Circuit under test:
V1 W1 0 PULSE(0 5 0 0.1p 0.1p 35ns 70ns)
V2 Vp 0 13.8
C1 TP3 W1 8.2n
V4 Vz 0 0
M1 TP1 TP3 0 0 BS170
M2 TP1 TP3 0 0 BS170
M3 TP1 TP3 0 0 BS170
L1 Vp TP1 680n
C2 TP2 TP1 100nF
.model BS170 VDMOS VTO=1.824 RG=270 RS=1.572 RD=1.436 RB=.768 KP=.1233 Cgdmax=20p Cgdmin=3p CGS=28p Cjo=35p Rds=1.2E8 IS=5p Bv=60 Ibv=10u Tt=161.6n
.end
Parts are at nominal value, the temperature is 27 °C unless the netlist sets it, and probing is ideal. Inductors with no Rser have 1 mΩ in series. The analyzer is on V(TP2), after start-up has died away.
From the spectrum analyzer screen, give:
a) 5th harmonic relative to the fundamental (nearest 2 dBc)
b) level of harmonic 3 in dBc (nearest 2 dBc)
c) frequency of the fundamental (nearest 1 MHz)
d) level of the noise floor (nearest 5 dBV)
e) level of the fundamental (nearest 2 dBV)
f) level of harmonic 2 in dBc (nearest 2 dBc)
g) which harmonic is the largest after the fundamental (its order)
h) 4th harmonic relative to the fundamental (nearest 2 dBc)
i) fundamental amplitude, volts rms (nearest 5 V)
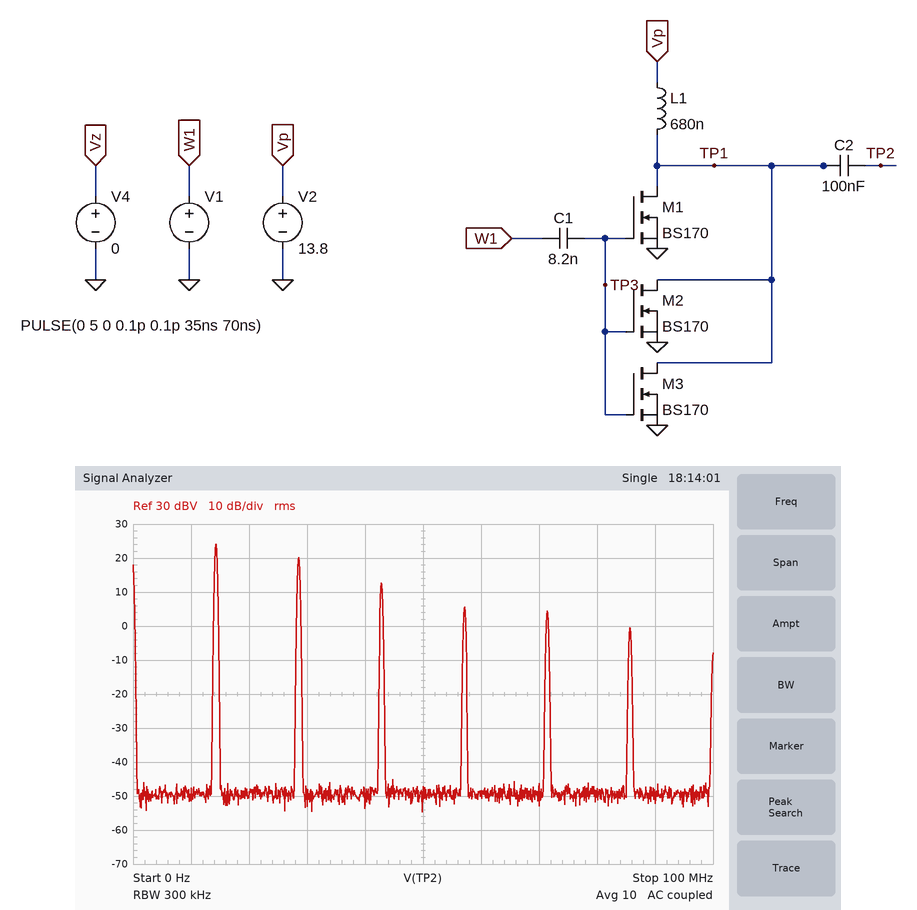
-20 dBc
-12 dBc
14 MHz
-50 dBV
24 dBV
-4 dBc
2
-18 dBc
15 V
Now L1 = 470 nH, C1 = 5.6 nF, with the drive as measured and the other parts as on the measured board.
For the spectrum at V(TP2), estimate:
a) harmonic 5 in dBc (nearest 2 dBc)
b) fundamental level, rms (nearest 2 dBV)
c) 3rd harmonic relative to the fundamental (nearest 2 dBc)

-18 dBc
24 dBV
-10 dBc
